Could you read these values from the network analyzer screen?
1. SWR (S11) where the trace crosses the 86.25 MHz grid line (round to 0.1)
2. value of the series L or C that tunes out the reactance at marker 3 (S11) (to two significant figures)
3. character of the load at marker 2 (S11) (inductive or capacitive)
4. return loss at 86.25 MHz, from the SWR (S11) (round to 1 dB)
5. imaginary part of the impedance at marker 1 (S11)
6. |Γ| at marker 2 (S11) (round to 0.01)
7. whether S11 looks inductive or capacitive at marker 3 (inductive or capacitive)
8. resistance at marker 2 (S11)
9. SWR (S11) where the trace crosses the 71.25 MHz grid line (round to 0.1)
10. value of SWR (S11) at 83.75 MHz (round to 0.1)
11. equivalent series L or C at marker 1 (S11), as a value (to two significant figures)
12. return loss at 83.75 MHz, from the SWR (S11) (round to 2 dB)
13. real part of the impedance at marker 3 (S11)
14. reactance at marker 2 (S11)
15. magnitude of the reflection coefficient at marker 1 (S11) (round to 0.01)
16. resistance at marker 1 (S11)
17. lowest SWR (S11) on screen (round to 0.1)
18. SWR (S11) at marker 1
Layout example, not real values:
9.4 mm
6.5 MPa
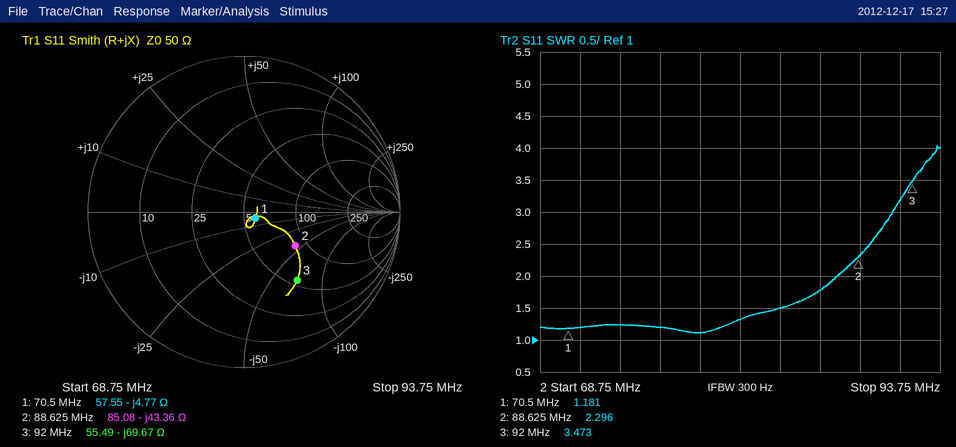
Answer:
1.8
120 nH
capacitive
11 dB
-4.77 Ω
0.39
capacitive
85.08 Ω
1.2
1.5
470 pF
14 dB
55.49 Ω
-43.36 Ω
0.08
57.55 Ω
1.1
1.181
